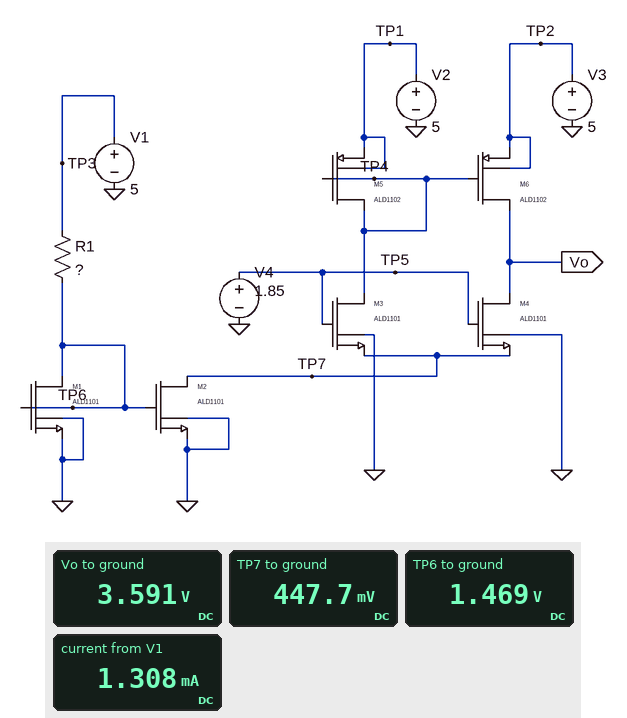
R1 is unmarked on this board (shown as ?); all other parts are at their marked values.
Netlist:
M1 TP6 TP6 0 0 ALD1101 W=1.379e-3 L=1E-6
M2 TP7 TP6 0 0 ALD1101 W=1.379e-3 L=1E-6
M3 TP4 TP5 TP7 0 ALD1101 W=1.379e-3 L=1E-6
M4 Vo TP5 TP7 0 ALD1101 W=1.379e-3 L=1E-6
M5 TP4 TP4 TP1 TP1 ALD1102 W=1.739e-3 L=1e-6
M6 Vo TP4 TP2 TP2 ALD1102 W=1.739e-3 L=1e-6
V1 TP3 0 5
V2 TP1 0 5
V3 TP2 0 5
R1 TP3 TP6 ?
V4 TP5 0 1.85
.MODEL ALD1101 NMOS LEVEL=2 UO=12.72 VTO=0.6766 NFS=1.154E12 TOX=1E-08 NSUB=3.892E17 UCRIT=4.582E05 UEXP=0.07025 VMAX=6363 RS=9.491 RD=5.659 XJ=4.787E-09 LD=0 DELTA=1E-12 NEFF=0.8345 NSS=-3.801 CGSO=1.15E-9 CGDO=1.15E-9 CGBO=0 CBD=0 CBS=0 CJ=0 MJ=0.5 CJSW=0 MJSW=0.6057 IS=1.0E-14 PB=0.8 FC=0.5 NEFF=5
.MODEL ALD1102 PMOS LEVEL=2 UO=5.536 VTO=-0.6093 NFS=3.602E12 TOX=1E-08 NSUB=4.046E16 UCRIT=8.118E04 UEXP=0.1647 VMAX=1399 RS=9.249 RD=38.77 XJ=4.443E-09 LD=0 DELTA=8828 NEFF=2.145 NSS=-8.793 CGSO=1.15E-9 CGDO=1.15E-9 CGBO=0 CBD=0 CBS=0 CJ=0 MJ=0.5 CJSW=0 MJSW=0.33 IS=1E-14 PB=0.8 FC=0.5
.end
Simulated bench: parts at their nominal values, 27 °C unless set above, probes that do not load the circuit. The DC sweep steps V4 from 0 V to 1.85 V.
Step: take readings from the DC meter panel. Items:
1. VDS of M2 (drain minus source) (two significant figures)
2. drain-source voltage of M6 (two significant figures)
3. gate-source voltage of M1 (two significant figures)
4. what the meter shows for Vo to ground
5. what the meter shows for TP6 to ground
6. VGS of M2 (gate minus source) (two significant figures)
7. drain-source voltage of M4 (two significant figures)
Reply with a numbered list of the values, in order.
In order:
1. 450 mV
2. -1.4 V
3. 1.5 V
4. 3.591 V
5. 1.469 V
6. 1.5 V
7. 3.1 V
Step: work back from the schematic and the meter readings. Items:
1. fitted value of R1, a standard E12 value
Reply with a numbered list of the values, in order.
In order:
1. 2.7 kΩ
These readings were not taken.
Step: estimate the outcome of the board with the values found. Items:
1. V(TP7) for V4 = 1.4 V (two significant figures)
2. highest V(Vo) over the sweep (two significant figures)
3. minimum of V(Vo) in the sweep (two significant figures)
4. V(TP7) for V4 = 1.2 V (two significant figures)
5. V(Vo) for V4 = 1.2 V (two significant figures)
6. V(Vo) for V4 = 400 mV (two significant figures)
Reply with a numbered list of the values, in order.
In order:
1. 210 mV
2. 5.0 V
3. 3.6 V
4. 130 mV
5. 3.9 V
6. 4.7 V
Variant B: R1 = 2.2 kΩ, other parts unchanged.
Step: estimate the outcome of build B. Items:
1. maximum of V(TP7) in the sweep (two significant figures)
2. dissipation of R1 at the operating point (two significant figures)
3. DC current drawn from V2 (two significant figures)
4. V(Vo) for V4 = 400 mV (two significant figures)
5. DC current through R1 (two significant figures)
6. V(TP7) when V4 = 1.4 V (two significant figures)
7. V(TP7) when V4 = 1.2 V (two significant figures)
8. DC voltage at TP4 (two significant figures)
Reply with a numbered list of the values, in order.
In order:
1. 420 mV
2. 5.4 mW
3. 690 µA
4. 4.7 V
5. 1.6 mA
6. 200 mV
7. 120 mV
8. 3.5 V
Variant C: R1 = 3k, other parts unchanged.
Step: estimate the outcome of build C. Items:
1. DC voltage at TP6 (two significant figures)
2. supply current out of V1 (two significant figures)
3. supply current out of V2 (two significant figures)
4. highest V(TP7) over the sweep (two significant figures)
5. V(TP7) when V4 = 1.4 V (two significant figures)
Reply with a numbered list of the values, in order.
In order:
1. 1.4 V
2. 1.2 mA
3. 570 µA
4. 460 mV
5. 220 mV
